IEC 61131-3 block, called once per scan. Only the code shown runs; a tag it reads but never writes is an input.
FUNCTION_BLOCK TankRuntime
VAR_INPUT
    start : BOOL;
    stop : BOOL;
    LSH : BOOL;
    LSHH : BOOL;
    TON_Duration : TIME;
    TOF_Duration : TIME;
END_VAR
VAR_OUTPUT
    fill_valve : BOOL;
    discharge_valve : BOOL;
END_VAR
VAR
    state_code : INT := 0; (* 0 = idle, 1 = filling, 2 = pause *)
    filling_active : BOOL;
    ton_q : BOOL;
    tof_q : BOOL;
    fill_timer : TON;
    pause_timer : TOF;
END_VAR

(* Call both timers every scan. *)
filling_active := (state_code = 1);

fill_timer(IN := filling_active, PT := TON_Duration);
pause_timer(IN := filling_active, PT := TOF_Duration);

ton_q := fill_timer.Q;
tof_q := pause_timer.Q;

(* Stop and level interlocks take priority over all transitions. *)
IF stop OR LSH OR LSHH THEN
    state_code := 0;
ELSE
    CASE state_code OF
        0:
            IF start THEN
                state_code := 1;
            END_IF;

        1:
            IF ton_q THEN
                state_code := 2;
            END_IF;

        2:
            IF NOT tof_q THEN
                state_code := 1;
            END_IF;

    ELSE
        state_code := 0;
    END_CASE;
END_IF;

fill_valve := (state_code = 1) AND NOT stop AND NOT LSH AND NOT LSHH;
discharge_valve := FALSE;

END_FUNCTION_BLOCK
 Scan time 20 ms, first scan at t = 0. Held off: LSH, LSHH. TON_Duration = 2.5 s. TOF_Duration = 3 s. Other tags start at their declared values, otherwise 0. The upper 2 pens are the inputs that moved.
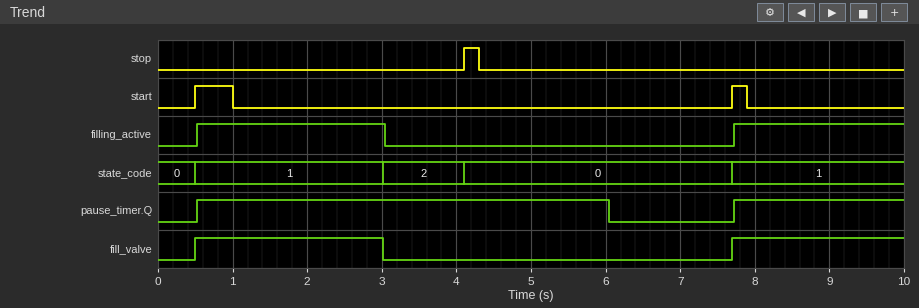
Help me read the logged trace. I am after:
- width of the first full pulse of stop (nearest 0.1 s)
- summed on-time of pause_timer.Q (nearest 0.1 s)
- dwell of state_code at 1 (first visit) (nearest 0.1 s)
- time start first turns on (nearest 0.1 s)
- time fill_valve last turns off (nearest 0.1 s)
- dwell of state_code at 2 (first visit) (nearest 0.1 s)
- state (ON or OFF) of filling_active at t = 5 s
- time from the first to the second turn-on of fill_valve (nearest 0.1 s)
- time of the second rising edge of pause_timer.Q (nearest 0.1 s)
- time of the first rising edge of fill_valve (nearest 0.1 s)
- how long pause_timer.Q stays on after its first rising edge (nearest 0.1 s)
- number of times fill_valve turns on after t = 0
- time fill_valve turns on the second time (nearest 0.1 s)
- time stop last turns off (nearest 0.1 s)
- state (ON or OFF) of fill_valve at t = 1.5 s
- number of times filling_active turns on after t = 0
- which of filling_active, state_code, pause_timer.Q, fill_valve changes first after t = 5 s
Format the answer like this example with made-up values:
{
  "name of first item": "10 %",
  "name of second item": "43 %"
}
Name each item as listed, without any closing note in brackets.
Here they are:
{
  "width of the first full pulse of stop": "0.2 s",
  "summed on-time of pause_timer.Q": "7.8 s",
  "dwell of state_code at 1 (first visit)": "2.5 s",
  "time start first turns on": "0.5 s",
  "time fill_valve last turns off": "3.0 s",
  "dwell of state_code at 2 (first visit)": "1.1 s",
  "state (ON or OFF) of filling_active at t = 5 s": "OFF",
  "time from the first to the second turn-on of fill_valve": "7.2 s",
  "time of the second rising edge of pause_timer.Q": "7.7 s",
  "time of the first rising edge of fill_valve": "0.5 s",
  "how long pause_timer.Q stays on after its first rising edge": "5.5 s",
  "number of times fill_valve turns on after t = 0": "2",
  "time fill_valve turns on the second time": "7.7 s",
  "time stop last turns off": "4.3 s",
  "state (ON or OFF) of fill_valve at t = 1.5 s": "ON",
  "number of times filling_active turns on after t = 0": "2",
  "which of filling_active, state_code, pause_timer.Q, fill_valve changes first after t = 5 s": "pause_timer.Q"
}
